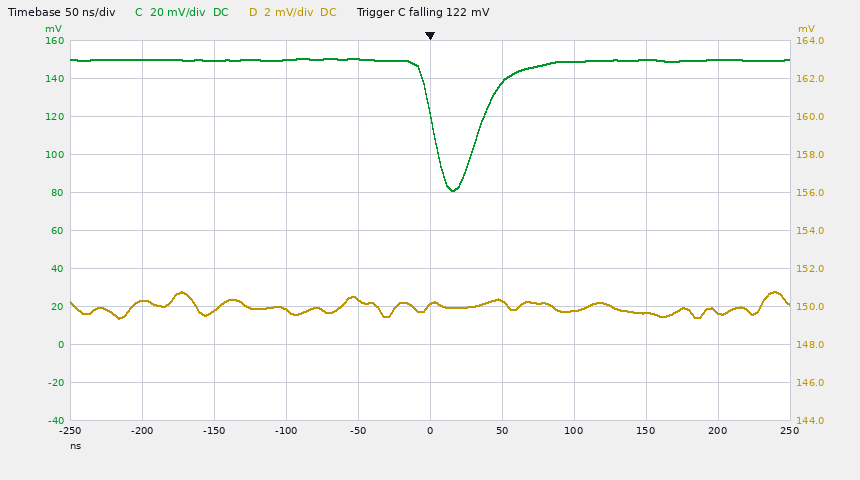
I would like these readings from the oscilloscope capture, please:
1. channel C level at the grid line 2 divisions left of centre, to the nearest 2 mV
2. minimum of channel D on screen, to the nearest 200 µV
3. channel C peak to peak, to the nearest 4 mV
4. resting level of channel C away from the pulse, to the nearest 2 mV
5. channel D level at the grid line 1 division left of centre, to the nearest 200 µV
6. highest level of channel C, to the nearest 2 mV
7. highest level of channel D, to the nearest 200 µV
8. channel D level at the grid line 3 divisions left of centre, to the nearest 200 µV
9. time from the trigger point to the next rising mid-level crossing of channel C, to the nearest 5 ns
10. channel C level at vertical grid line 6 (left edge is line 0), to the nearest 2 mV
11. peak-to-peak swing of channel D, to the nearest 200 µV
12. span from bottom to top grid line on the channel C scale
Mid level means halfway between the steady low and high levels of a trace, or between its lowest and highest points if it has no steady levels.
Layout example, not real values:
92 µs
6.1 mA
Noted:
150 mV
149.4 mV
68 mV
150 mV
150.4 mV
150 mV
150.8 mV
149.8 mV
35 ns
138 mV
1.4 mV
200 mV
